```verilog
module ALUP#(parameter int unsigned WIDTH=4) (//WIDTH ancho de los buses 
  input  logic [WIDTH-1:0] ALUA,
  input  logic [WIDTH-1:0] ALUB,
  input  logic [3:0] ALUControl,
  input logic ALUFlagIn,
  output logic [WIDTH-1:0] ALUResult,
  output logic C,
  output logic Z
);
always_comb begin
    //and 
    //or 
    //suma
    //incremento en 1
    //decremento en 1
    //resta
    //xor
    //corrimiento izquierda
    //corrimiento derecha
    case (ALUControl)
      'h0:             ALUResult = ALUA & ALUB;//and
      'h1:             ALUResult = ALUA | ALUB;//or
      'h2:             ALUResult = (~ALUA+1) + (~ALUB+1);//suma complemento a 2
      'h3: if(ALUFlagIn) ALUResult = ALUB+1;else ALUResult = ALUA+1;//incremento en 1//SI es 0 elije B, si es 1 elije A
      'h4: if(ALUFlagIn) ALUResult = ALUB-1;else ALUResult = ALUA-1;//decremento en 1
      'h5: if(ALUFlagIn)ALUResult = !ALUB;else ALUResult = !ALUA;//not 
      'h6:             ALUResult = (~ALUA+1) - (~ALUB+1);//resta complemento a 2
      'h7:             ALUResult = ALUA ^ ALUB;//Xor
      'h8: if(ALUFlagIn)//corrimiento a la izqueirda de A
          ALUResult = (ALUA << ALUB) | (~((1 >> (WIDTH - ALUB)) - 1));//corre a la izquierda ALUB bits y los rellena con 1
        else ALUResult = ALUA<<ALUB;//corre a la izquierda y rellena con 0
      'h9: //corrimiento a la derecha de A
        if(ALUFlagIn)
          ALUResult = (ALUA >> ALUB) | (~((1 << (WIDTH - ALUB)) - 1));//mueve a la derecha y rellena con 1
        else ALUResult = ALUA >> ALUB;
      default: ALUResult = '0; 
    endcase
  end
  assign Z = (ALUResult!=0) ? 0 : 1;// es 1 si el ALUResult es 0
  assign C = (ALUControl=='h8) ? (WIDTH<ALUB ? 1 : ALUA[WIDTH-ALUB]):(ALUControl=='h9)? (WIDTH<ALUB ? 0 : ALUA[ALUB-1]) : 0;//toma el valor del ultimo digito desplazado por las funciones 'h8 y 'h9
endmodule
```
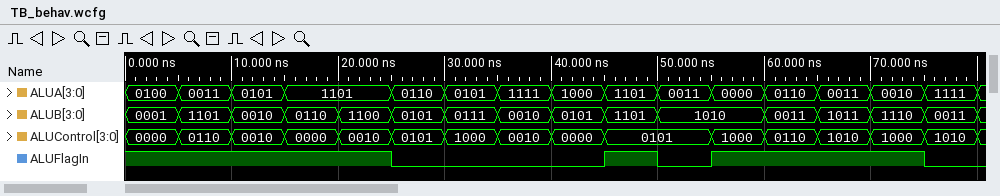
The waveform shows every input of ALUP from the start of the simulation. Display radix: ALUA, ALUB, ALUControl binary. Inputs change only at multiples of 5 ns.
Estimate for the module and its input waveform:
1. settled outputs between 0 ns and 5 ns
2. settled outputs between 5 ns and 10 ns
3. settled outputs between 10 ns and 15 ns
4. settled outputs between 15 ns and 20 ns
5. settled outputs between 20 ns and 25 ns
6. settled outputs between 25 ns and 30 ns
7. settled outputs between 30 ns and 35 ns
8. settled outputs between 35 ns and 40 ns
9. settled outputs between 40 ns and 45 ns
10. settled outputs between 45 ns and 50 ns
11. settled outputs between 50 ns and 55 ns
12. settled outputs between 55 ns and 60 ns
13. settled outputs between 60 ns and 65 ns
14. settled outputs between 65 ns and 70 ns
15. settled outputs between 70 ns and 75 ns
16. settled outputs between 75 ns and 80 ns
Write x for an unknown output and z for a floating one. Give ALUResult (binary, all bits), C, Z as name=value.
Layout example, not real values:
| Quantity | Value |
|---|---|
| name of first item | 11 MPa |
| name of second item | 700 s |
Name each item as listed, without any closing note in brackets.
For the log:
| Quantity | Value |
|---|---|
| settled outputs between 0 ns and 5 ns | ALUResult=0000, C=0, Z=1 |
| settled outputs between 5 ns and 10 ns | ALUResult=1010, C=0, Z=0 |
| settled outputs between 10 ns and 15 ns | ALUResult=1001, C=0, Z=0 |
| settled outputs between 15 ns and 20 ns | ALUResult=0100, C=0, Z=0 |
| settled outputs between 20 ns and 25 ns | ALUResult=0111, C=0, Z=0 |
| settled outputs between 25 ns and 30 ns | ALUResult=0000, C=0, Z=1 |
| settled outputs between 30 ns and 35 ns | ALUResult=0000, C=1, Z=1 |
| settled outputs between 35 ns and 40 ns | ALUResult=1111, C=0, Z=0 |
| settled outputs between 40 ns and 45 ns | ALUResult=0000, C=0, Z=1 |
| settled outputs between 45 ns and 50 ns | ALUResult=0000, C=0, Z=1 |
| settled outputs between 50 ns and 55 ns | ALUResult=0000, C=0, Z=1 |
| settled outputs between 55 ns and 60 ns | ALUResult=0000, C=1, Z=1 |
| settled outputs between 60 ns and 65 ns | ALUResult=1101, C=0, Z=0 |
| settled outputs between 65 ns and 70 ns | ALUResult=0000, C=0, Z=1 |
| settled outputs between 70 ns and 75 ns | ALUResult=0000, C=1, Z=1 |
| settled outputs between 75 ns and 80 ns | ALUResult=0000, C=0, Z=1 |
